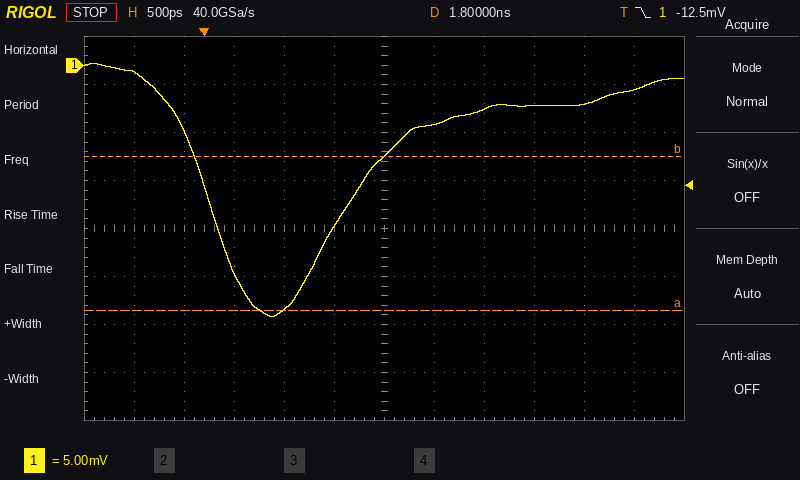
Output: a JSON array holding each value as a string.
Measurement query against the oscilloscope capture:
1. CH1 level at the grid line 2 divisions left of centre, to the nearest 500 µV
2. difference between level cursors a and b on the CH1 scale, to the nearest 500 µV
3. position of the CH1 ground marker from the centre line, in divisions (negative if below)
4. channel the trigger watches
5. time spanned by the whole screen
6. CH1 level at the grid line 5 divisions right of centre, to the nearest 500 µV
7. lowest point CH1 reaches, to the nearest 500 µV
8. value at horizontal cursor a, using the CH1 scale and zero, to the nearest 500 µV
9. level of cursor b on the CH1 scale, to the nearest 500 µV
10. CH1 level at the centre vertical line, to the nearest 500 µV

["-25.5 mV", "16.0 mV", "+3.4 div", "CH1", "6 ns", "-2.5 mV", "-26.0 mV", "-25.5 mV", "-9.5 mV", "-9.5 mV"]
